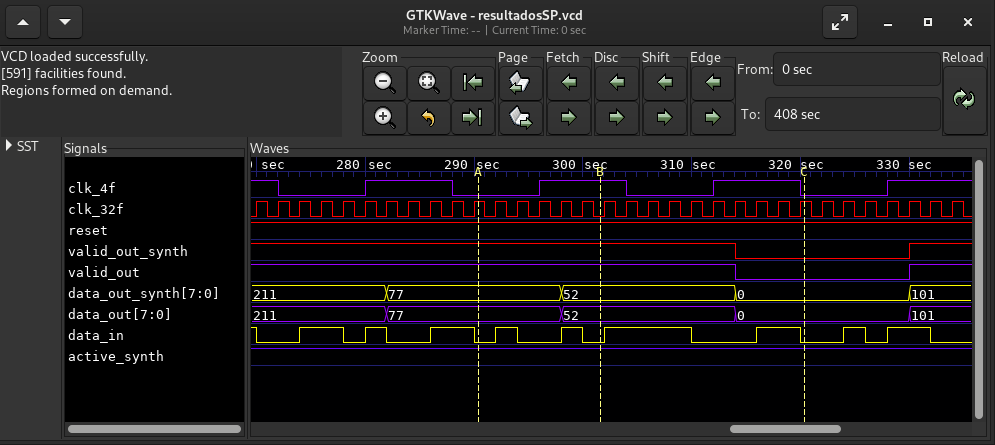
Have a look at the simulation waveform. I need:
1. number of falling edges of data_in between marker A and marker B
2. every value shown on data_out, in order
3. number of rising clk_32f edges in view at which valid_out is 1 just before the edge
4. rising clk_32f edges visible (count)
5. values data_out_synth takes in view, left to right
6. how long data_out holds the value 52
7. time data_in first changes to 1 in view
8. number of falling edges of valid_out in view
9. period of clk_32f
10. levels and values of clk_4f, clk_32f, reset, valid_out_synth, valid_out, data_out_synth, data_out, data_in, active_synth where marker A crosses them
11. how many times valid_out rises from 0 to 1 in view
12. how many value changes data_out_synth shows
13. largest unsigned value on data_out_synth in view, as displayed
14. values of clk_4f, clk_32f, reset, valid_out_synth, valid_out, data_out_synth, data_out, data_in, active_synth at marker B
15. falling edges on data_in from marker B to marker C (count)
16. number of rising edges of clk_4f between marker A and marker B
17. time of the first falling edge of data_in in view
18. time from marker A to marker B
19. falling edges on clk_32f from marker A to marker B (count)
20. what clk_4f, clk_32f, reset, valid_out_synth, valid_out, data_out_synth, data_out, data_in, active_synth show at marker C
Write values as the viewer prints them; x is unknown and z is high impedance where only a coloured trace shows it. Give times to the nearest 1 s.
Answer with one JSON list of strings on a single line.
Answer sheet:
["2", "211, 77, 52, 0, 101", "25", "33", "211, 77, 52, 0, 101", "16 s", "274 s", "1", "2 s", "clk_4f=0, clk_32f=1, reset=1, valid_out_synth=1, valid_out=1, data_out_synth=77, data_out=77, data_in=0, active_synth=1", "1", "4", "211", "clk_4f=1, clk_32f=0, reset=1, valid_out_synth=1, valid_out=1, data_out_synth=52, data_out=52, data_in=0, active_synth=1", "2", "1", "270 s", "11 s", "6", "clk_4f=0, clk_32f=1, reset=1, valid_out_synth=0, valid_out=0, data_out_synth=0, data_out=0, data_in=0, active_synth=1"]
